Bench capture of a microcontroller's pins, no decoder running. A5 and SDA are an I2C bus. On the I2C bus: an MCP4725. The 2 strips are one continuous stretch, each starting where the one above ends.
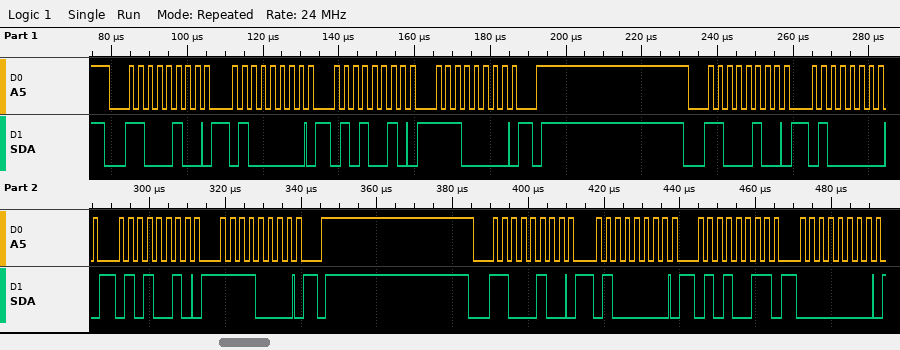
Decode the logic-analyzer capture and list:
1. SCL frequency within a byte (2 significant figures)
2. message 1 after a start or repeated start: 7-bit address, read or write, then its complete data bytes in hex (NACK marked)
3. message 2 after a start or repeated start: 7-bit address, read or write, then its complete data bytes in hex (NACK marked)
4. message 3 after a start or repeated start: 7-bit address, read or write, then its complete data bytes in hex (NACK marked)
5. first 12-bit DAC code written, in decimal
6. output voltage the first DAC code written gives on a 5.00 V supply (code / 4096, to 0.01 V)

400 kHz
0x62 write: 40 52 E0
0x62 write: 40 52 F0
0x62 write: 40 53 00
1326
1.62 V
